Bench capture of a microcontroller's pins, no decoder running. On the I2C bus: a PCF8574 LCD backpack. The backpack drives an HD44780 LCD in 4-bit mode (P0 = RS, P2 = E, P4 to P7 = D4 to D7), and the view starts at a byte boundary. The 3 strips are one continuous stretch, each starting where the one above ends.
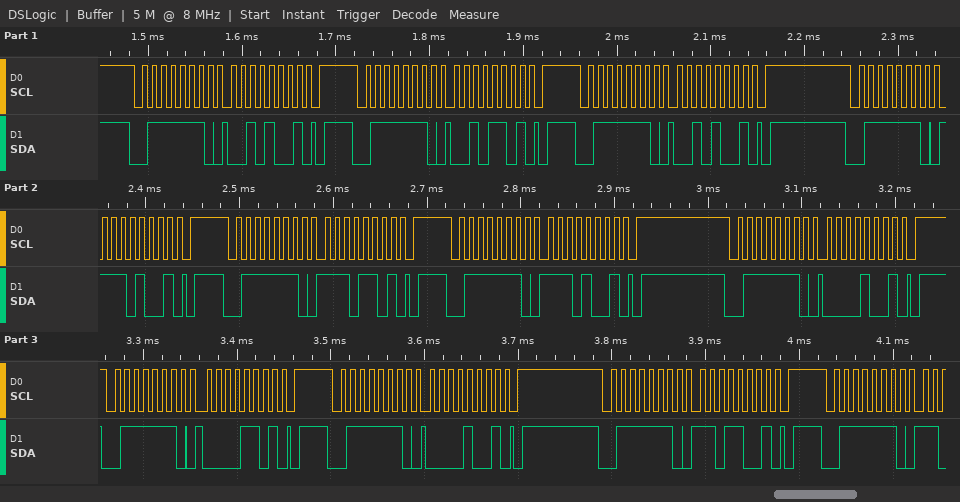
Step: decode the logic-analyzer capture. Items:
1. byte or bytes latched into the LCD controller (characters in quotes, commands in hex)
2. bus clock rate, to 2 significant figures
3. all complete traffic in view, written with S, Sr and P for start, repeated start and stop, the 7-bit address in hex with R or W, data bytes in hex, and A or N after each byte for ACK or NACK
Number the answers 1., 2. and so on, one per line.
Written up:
1. '.'
2. 100 kHz
3. S 3FW A 29 A P S 3FW A 2D A P S 3FW A 29 A P S 3FW A E9 A P S 3FW A ED A P S 3FW A E9 A P S 3FW A 09 A P S 3FW A 0D A P S 3FW A 09 A P S 3FW A D9 A P S 3FW A
